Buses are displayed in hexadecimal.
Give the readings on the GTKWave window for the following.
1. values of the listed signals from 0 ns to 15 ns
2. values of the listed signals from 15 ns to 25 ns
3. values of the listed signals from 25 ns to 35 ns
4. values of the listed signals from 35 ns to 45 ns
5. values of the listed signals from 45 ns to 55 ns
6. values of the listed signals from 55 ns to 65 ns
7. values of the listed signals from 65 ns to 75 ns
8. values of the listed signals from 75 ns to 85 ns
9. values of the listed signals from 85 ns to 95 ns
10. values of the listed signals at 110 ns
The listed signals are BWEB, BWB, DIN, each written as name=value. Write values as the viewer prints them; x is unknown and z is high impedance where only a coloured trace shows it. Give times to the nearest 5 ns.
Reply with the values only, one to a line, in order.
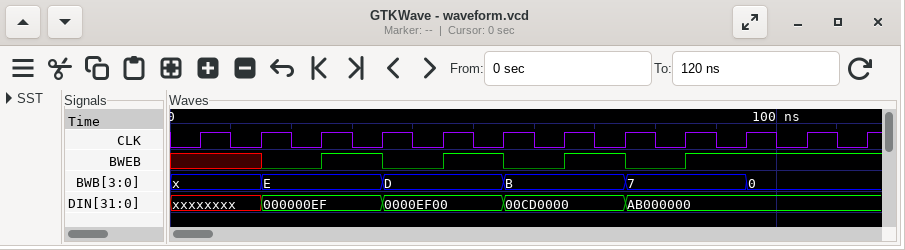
BWEB=x, BWB=x, DIN=xxxxxxxx
BWEB=0, BWB=E, DIN=000000EF
BWEB=1, BWB=E, DIN=000000EF
BWEB=0, BWB=D, DIN=0000EF00
BWEB=1, BWB=D, DIN=0000EF00
BWEB=0, BWB=B, DIN=00CD0000
BWEB=1, BWB=B, DIN=00CD0000
BWEB=0, BWB=7, DIN=AB000000
BWEB=1, BWB=7, DIN=AB000000
BWEB=1, BWB=0, DIN=AB000000
